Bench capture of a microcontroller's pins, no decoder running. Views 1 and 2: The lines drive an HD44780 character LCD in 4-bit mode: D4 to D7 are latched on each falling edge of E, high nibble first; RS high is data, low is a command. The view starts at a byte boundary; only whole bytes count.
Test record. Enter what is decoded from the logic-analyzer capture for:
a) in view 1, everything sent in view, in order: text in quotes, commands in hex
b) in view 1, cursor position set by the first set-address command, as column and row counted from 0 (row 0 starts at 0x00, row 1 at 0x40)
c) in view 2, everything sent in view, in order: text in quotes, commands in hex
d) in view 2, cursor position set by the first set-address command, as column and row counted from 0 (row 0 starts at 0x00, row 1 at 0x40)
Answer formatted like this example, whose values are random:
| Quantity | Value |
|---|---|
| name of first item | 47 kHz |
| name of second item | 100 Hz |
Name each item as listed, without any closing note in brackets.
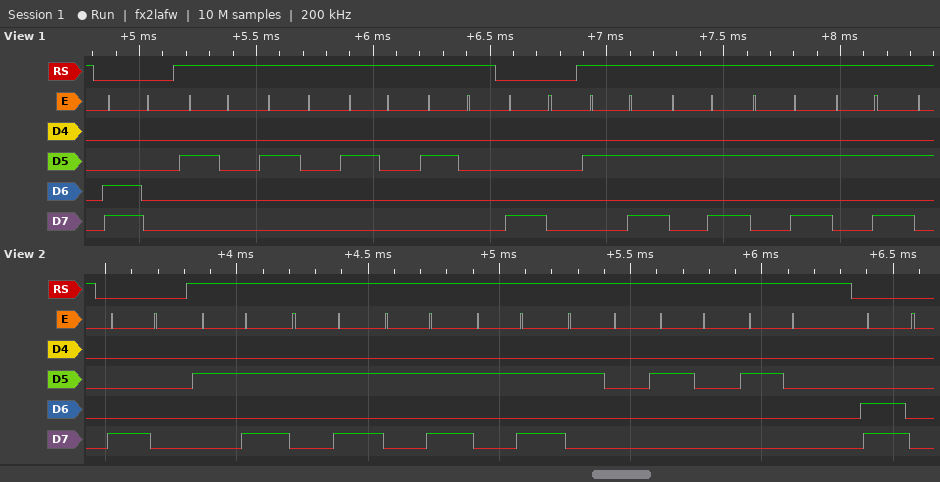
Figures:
| Quantity | Value |
|---|---|
| in view 1, everything sent in view, in order: text in quotes, commands in hex | 0xC0 "    " 0x80 "****" |
| in view 1, cursor position set by the first set-address command, as column and row counted from 0 | column 0, row 1 |
| in view 2, everything sent in view, in order: text in quotes, commands in hex | 0x80 "****   " 0xC0 |
| in view 2, cursor position set by the first set-address command, as column and row counted from 0 | column 0, row 0 |
